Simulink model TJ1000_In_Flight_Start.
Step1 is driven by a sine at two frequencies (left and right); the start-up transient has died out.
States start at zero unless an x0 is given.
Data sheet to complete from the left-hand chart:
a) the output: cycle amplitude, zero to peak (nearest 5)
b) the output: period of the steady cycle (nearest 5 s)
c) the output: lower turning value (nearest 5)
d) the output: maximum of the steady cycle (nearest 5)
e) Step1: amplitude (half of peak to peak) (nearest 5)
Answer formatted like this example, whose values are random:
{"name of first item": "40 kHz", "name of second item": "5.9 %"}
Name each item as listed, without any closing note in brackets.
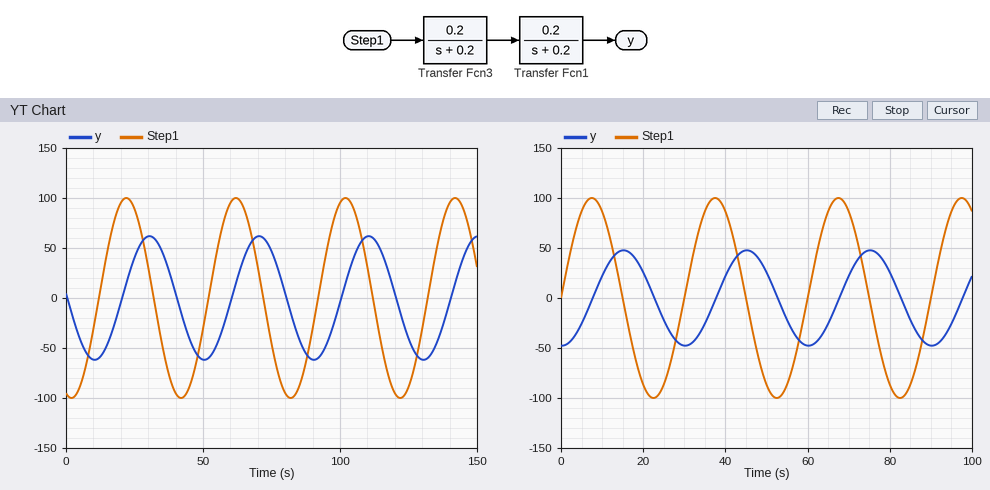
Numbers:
{"the output: cycle amplitude, zero to peak": "60", "the output: period of the steady cycle": "40 s", "the output: lower turning value": "-60", "the output: maximum of the steady cycle": "60", "Step1: amplitude (half of peak to peak)": "100"}
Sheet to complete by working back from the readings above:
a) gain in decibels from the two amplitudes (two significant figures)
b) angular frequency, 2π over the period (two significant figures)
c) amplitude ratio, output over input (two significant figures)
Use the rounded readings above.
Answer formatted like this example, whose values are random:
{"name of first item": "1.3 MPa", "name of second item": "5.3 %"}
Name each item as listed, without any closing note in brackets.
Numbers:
{"gain in decibels from the two amplitudes": "-4.4 dB", "angular frequency, 2π over the period": "0.16 rad/s", "amplitude ratio, output over input": "0.60"}
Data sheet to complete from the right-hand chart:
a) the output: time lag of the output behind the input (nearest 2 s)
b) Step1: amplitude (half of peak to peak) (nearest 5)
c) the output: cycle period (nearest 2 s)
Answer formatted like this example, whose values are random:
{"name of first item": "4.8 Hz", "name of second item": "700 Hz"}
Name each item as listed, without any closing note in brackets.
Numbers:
{"the output: time lag of the output behind the input": "8 s", "Step1: amplitude (half of peak to peak)": "100", "the output: cycle period": "30 s"}
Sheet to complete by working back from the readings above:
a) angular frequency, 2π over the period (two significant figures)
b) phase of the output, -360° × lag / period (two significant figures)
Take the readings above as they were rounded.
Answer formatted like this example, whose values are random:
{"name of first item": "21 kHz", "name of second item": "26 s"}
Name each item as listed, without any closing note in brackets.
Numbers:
{"angular frequency, 2π over the period": "0.21 rad/s", "phase of the output, -360° × lag / period": "-96°"}
